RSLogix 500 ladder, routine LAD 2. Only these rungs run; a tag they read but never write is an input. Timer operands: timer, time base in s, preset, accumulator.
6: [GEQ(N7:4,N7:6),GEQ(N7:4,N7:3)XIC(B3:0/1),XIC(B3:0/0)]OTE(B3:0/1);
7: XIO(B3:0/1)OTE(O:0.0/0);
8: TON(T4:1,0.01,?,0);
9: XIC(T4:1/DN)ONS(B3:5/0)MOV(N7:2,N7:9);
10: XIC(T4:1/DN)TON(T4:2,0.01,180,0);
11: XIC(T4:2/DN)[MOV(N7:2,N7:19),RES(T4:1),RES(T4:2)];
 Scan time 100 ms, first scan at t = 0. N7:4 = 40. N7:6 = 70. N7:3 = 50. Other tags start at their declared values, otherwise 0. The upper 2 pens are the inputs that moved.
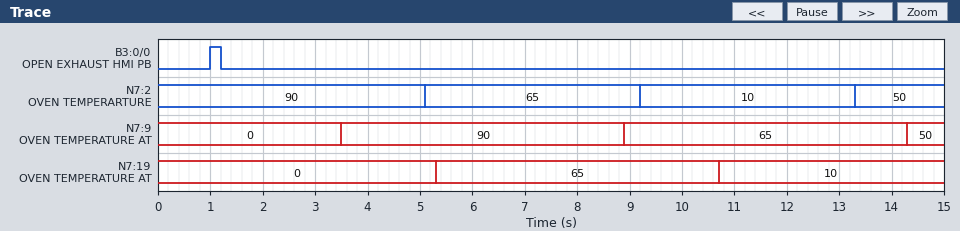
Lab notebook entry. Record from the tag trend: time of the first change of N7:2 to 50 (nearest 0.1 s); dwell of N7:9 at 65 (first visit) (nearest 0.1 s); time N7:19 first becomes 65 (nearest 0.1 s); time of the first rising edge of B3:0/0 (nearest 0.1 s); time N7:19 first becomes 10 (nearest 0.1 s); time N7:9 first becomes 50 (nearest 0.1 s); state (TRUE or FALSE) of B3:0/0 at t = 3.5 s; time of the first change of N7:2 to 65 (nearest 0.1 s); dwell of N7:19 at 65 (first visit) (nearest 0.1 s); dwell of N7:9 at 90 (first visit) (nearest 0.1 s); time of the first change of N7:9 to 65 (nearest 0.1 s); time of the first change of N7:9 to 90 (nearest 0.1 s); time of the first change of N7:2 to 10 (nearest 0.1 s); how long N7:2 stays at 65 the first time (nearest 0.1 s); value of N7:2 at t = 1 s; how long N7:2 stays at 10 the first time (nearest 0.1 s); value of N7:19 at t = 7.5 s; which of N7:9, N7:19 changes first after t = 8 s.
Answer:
13.3 s
5.4 s
5.3 s
1.0 s
10.7 s
14.3 s
FALSE
5.1 s
5.4 s
5.4 s
8.9 s
3.5 s
9.2 s
4.1 s
90
4.1 s
65
N7:9
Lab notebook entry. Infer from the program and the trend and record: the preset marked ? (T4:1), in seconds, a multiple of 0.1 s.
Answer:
3.5 s
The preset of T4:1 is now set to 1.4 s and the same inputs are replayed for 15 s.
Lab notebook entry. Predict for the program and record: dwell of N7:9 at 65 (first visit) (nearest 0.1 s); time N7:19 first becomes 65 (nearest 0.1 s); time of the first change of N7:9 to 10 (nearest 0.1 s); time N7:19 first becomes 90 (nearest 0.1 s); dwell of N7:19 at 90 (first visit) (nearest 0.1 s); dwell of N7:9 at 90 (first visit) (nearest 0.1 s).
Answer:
3.3 s
6.5 s
11.3 s
3.2 s
3.3 s
6.6 s
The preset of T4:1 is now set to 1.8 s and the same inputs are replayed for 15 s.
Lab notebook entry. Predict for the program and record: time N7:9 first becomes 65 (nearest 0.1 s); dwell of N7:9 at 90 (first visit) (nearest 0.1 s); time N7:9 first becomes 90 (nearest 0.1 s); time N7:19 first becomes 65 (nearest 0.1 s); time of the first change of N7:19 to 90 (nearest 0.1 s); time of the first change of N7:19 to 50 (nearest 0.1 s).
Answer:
5.5 s
3.7 s
1.8 s
7.3 s
3.6 s
14.7 s
